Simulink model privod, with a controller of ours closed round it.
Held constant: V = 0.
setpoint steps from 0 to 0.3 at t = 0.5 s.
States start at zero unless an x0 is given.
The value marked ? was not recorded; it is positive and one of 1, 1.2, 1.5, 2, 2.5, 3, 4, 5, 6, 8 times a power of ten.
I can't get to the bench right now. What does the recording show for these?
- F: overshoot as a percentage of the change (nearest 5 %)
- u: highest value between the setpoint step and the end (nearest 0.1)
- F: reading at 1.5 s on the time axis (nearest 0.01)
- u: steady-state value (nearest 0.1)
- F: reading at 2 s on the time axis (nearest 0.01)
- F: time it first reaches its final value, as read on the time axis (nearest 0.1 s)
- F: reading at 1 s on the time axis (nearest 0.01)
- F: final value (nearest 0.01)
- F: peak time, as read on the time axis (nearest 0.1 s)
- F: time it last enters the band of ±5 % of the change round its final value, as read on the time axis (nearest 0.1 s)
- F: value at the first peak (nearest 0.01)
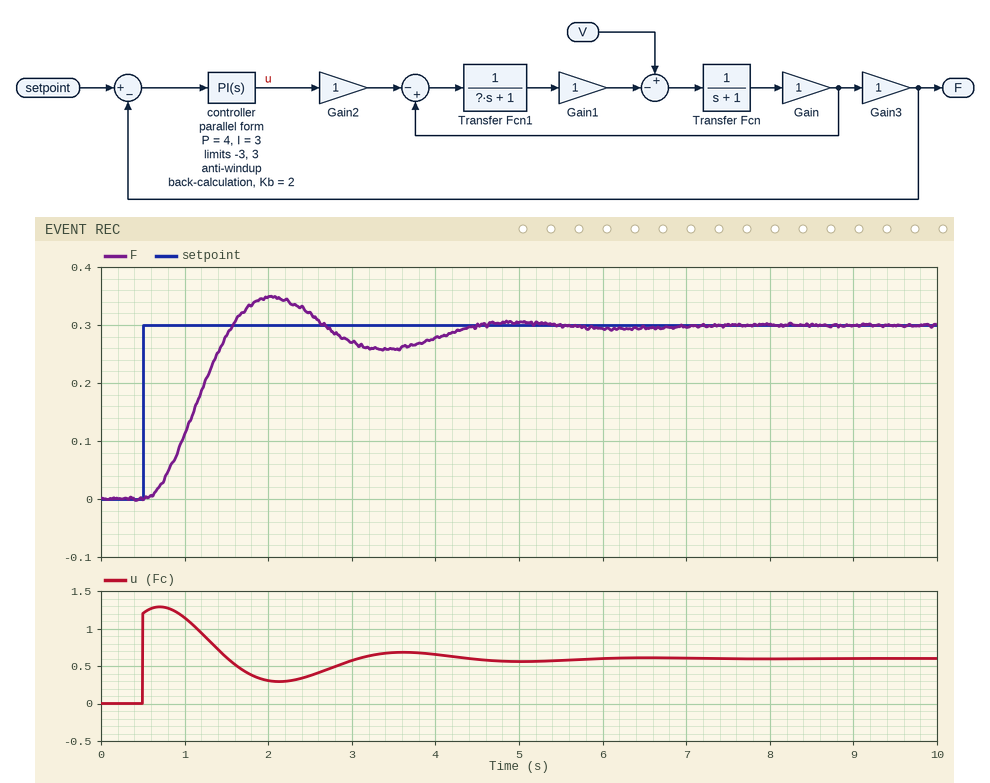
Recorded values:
15 %
1.3
0.28
0.6
0.35
1.6 s
0.11
0.30
2.0 s
4.2 s
0.35
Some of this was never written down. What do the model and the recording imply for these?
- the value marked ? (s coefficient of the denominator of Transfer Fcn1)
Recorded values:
1
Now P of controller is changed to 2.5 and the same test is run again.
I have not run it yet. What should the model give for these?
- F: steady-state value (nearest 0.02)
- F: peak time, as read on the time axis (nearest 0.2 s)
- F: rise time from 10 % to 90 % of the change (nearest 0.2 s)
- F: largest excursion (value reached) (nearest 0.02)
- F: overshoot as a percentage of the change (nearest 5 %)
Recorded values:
0.30
2.4 s
0.8 s
0.36
20 %
